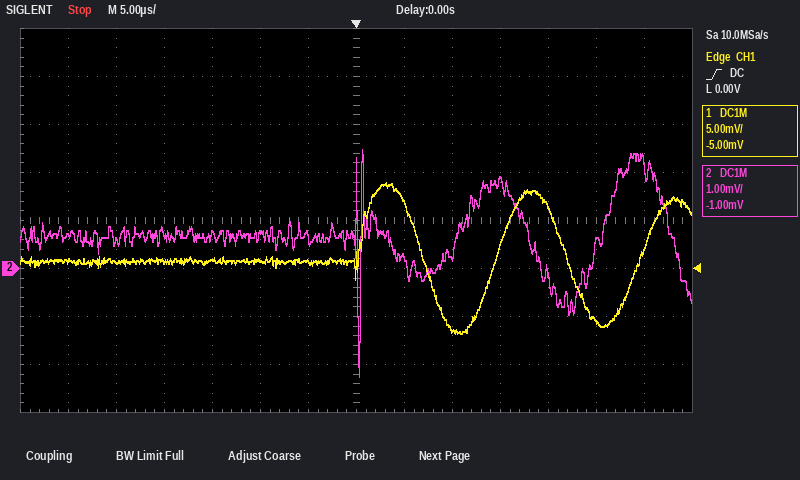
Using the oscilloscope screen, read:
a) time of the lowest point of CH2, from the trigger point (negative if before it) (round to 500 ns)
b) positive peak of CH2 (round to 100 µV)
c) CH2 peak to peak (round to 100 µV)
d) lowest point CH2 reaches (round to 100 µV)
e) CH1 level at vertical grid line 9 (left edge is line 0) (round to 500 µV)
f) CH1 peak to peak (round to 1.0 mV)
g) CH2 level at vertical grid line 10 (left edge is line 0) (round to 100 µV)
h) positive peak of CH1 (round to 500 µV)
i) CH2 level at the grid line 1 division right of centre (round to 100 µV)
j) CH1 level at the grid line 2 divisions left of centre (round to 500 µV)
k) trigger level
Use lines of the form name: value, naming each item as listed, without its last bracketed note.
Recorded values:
time of the lowest point of CH2, from the trigger point (negative if before it): +500 ns
positive peak of CH2: 2.5 mV
CH2 peak to peak: 4.7 mV
lowest point CH2 reaches: -2.2 mV
CH1 level at vertical grid line 9 (left edge is line 0): -6.5 mV
CH1 peak to peak: 16.0 mV
CH2 level at vertical grid line 10 (left edge is line 0): 1.8 mV
positive peak of CH1: 9.0 mV
CH2 level at the grid line 1 division right of centre: 200 µV
CH1 level at the grid line 2 divisions left of centre: 1.0 mV
trigger level: 0.00 V
